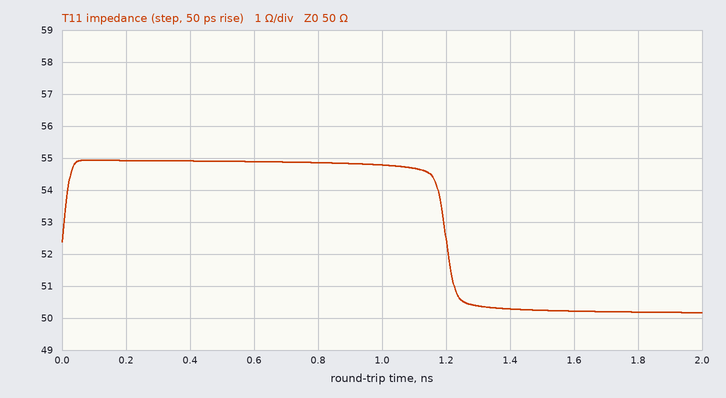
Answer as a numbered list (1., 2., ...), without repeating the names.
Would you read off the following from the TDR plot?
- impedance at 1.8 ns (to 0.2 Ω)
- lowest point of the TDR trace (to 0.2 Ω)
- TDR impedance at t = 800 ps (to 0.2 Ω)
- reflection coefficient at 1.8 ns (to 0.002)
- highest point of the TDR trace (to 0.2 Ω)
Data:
1. 50.2 Ω
2. 50.2 Ω
3. 54.8 Ω
4. +0.002
5. 55.0 Ω
